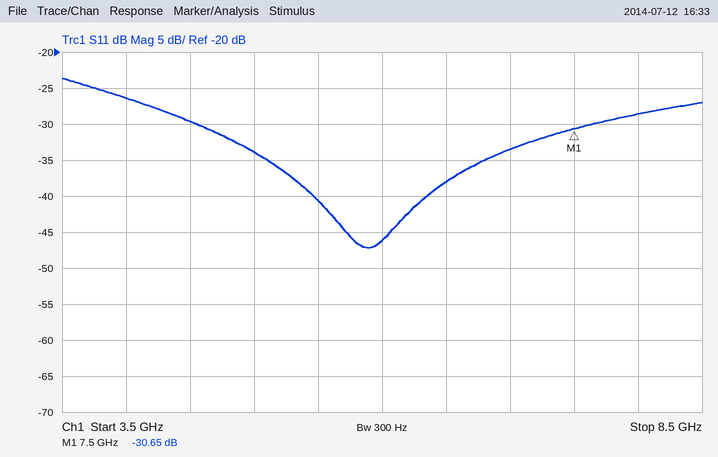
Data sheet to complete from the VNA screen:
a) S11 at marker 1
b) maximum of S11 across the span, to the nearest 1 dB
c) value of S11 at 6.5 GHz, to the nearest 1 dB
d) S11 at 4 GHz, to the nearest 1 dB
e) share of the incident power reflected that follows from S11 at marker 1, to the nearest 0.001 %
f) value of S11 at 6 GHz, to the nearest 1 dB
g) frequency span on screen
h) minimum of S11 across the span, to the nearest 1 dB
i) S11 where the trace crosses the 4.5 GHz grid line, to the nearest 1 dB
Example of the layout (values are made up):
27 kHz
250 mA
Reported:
-30.65 dB
-24 dB
-38 dB
-26 dB
0.086 %
-46 dB
5 GHz
-47 dB
-30 dB
